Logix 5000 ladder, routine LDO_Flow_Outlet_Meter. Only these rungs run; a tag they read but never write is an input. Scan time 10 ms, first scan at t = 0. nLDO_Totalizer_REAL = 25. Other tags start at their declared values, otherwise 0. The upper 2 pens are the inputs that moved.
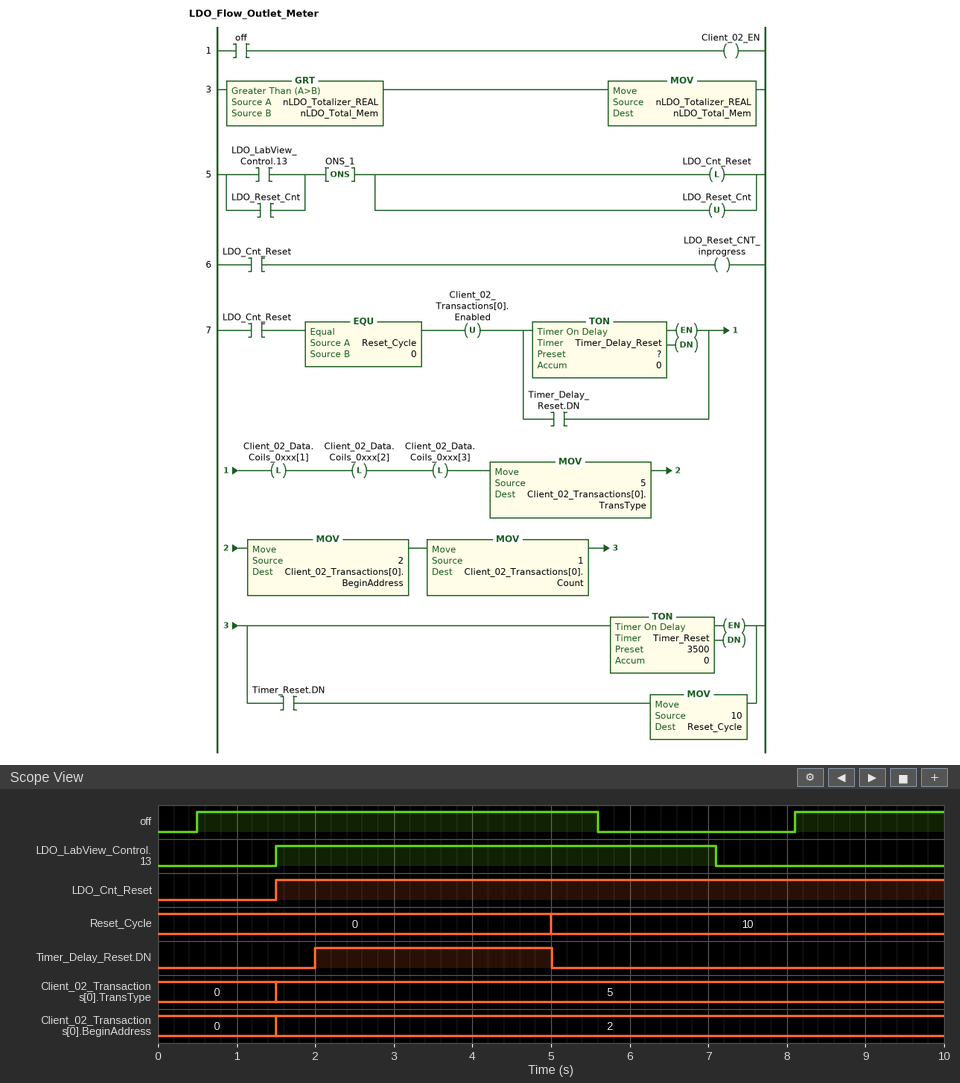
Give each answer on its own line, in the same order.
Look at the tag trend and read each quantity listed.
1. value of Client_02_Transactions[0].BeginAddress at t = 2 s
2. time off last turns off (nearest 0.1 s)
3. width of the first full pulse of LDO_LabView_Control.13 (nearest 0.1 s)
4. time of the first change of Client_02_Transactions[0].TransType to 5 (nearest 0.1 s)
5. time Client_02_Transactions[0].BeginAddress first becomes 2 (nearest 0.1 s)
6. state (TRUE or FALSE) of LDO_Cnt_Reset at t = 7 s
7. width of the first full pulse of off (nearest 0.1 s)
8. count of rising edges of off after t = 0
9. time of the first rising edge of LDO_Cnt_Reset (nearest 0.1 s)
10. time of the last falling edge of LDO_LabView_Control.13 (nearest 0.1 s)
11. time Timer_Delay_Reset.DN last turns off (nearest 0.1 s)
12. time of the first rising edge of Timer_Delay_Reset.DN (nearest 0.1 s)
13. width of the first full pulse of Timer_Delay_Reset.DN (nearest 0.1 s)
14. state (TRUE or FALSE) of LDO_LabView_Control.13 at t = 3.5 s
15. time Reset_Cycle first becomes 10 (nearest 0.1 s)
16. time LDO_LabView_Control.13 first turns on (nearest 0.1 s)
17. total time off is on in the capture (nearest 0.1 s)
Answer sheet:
2
5.6 s
5.6 s
1.5 s
1.5 s
TRUE
5.1 s
2
1.5 s
7.1 s
5.0 s
2.0 s
3.0 s
TRUE
5.0 s
1.5 s
7.0 s
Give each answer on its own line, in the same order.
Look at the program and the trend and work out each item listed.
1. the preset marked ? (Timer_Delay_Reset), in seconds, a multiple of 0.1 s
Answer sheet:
0.5 s
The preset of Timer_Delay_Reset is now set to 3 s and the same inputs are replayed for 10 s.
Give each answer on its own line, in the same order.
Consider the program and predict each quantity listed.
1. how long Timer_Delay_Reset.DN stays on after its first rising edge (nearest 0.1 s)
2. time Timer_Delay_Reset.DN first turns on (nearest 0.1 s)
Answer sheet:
0.5 s
4.5 s
